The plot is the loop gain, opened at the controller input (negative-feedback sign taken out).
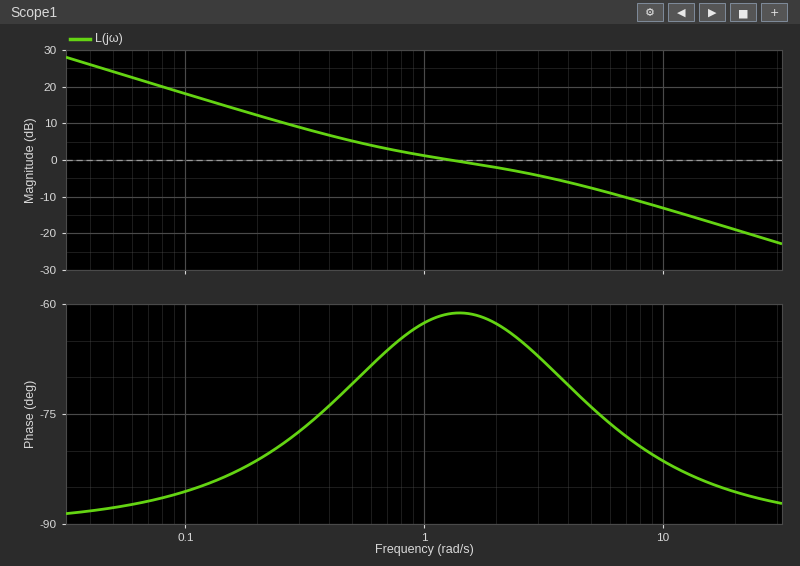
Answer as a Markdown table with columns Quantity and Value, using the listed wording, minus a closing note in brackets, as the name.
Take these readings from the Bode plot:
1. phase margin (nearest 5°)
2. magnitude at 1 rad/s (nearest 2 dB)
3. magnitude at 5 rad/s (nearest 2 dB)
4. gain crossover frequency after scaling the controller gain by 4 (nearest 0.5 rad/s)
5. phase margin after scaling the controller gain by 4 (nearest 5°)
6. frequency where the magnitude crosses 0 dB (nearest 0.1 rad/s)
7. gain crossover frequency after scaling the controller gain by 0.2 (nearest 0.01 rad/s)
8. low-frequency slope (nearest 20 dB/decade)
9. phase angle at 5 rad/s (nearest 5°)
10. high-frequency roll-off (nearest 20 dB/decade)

| Quantity | Value |
|---|---|
| phase margin | 120° |
| magnitude at 1 rad/s | 2 dB |
| magnitude at 5 rad/s | -8 dB |
| gain crossover frequency after scaling the controller gain by 4 | 9.0 rad/s |
| phase margin after scaling the controller gain by 4 | 100° |
| frequency where the magnitude crosses 0 dB | 1.3 rad/s |
| gain crossover frequency after scaling the controller gain by 0.2 | 0.16 rad/s |
| low-frequency slope | -20 dB/decade |
| phase angle at 5 rad/s | -75° |
| high-frequency roll-off | -20 dB/decade |
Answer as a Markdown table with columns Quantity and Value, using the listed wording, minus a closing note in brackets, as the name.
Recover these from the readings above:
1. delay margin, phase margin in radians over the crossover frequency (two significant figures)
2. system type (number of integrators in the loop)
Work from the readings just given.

| Quantity | Value |
|---|---|
| delay margin, phase margin in radians over the crossover frequency | 1.6 s |
| system type | 1 |
